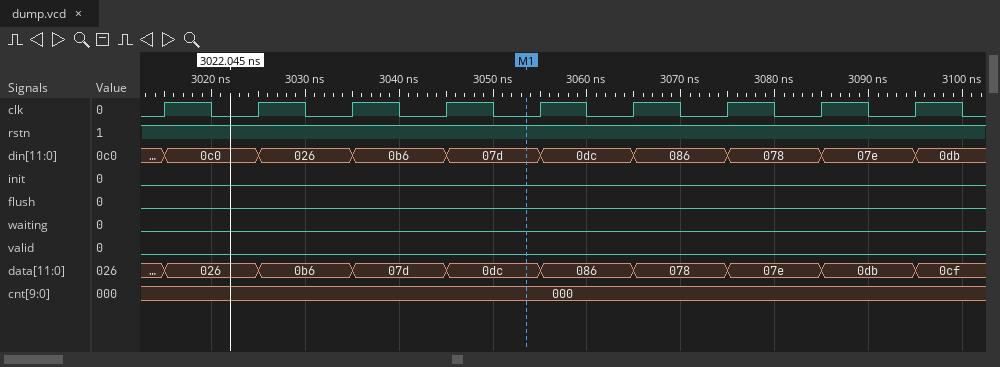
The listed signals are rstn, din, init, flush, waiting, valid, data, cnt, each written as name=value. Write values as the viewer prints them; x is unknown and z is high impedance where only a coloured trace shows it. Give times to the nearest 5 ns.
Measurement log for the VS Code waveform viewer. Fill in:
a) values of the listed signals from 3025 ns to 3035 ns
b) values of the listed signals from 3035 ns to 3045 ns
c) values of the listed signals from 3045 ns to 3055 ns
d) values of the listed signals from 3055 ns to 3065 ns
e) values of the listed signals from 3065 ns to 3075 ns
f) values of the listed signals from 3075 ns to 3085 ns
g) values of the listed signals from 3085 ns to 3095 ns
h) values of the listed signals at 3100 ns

rstn=1, din=026, init=0, flush=0, waiting=0, valid=0, data=0b6, cnt=000
rstn=1, din=0b6, init=0, flush=0, waiting=0, valid=0, data=07d, cnt=000
rstn=1, din=07d, init=0, flush=0, waiting=0, valid=0, data=0dc, cnt=000
rstn=1, din=0dc, init=0, flush=0, waiting=0, valid=0, data=086, cnt=000
rstn=1, din=086, init=0, flush=0, waiting=0, valid=0, data=078, cnt=000
rstn=1, din=078, init=0, flush=0, waiting=0, valid=0, data=07e, cnt=000
rstn=1, din=07e, init=0, flush=0, waiting=0, valid=0, data=0db, cnt=000
rstn=1, din=0db, init=0, flush=0, waiting=0, valid=0, data=0cf, cnt=000
